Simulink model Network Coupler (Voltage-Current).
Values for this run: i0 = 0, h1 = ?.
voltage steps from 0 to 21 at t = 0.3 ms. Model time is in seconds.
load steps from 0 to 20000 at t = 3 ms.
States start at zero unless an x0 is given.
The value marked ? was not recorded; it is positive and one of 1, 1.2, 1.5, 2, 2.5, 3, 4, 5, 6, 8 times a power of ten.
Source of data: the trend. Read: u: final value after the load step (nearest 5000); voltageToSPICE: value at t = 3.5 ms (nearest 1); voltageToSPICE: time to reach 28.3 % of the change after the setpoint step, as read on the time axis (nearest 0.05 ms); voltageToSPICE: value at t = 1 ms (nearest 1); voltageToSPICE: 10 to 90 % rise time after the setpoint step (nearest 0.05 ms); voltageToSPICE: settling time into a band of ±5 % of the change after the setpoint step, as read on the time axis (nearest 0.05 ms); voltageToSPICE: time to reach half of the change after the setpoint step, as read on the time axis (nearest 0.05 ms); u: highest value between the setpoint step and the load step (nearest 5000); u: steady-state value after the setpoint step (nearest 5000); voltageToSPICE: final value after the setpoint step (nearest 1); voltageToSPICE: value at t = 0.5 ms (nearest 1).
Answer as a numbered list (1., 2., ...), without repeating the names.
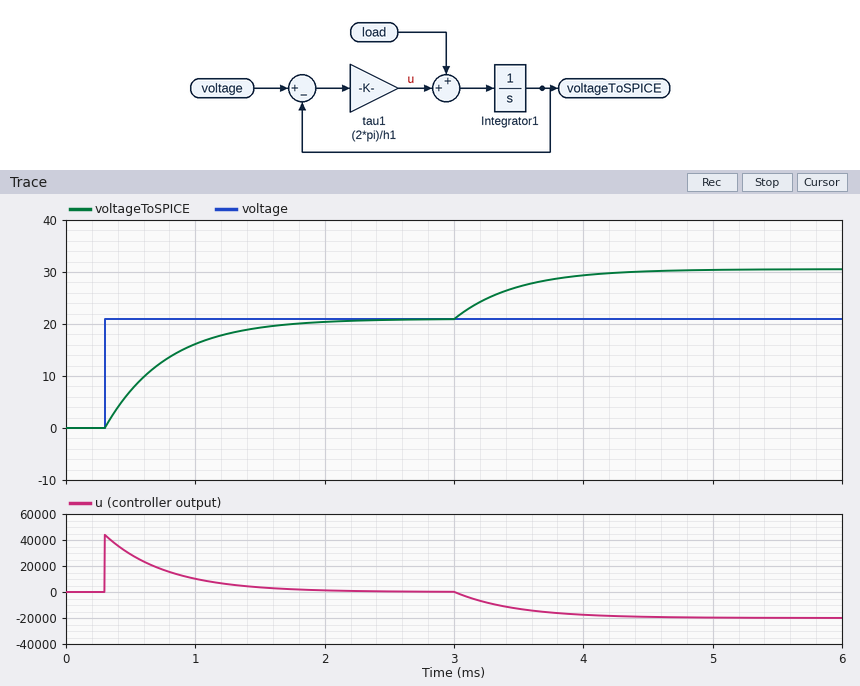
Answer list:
1. -20000
2. 27
3. 0.45 ms
4. 16
5. 1.05 ms
6. 1.75 ms
7. 0.65 ms
8. 45000
9. 0
10. 21
11. 7
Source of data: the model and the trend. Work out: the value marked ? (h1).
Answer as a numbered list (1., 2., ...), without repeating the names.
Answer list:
1. 0.003
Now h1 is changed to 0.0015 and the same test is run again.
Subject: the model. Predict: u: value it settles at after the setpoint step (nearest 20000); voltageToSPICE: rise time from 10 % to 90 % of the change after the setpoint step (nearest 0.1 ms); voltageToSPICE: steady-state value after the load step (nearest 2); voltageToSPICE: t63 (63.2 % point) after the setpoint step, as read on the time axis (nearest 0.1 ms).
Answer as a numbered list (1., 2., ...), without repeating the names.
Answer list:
1. 0
2. 0.5 ms
3. 26
4. 0.5 ms
